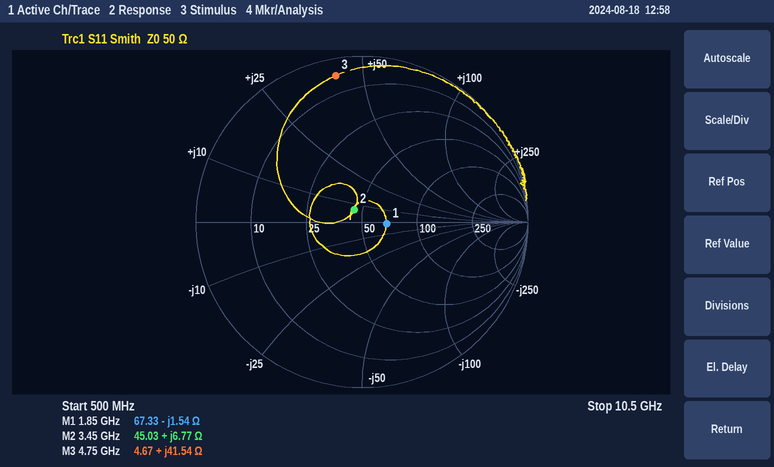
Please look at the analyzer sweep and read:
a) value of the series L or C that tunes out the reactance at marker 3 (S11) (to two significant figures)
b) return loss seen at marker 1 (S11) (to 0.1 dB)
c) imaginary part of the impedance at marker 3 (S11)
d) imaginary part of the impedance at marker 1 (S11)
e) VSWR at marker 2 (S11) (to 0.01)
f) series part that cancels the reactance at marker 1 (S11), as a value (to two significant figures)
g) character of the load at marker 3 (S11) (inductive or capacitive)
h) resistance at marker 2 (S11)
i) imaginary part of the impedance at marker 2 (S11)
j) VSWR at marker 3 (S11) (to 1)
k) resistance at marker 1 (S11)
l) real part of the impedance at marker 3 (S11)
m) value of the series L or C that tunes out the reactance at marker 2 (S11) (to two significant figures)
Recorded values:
810 fF
16.6 dB
+41.54 Ω
-1.54 Ω
1.19
130 pH
inductive
45.03 Ω
+6.77 Ω
18
67.33 Ω
4.67 Ω
6.8 pF
